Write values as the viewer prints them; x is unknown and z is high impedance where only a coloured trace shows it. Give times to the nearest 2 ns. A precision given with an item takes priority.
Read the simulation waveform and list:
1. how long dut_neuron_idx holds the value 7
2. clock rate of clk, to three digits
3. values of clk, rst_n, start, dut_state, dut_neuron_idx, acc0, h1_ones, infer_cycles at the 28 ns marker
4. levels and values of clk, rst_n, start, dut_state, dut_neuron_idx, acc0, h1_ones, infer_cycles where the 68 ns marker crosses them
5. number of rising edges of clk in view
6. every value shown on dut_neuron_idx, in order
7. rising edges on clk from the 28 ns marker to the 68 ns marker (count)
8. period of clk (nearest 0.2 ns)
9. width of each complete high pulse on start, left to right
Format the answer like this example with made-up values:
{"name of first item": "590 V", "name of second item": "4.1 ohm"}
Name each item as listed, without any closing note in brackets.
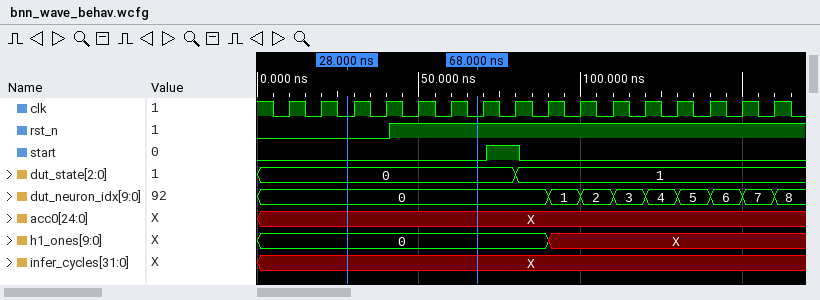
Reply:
{"how long dut_neuron_idx holds the value 7": "10 ns", "clock rate of clk, to three digits": "100 MHz", "values of clk, rst_n, start, dut_state, dut_neuron_idx, acc0, h1_ones, infer_cycles at the 28 ns marker": "clk=0, rst_n=0, start=0, dut_state=0, dut_neuron_idx=0, acc0=X, h1_ones=0, infer_cycles=X", "levels and values of clk, rst_n, start, dut_state, dut_neuron_idx, acc0, h1_ones, infer_cycles where the 68 ns marker crosses them": "clk=0, rst_n=1, start=0, dut_state=0, dut_neuron_idx=0, acc0=X, h1_ones=0, infer_cycles=X", "number of rising edges of clk in view": "16", "every value shown on dut_neuron_idx, in order": "0, 1, 2, 3, 4, 5, 6, 7, 8", "rising edges on clk from the 28 ns marker to the 68 ns marker": "4", "period of clk": "10 ns", "width of each complete high pulse on start, left to right": "10 ns"}
